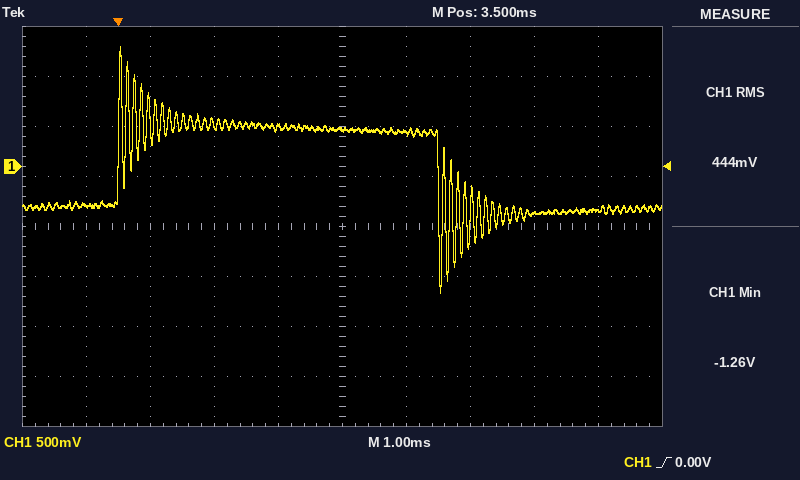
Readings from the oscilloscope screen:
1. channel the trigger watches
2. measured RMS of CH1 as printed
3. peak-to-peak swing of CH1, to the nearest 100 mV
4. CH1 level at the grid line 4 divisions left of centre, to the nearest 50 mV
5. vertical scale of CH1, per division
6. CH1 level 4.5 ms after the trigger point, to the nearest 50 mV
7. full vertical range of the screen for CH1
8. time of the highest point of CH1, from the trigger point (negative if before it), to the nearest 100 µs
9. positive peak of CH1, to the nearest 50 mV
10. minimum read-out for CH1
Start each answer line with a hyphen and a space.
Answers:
- CH1
- 444 mV
- 2.50 V
- -400 mV
- 500 mV
- 350 mV
- 4 V
- 0.0 ms
- 1.20 V
- -1.26 V
